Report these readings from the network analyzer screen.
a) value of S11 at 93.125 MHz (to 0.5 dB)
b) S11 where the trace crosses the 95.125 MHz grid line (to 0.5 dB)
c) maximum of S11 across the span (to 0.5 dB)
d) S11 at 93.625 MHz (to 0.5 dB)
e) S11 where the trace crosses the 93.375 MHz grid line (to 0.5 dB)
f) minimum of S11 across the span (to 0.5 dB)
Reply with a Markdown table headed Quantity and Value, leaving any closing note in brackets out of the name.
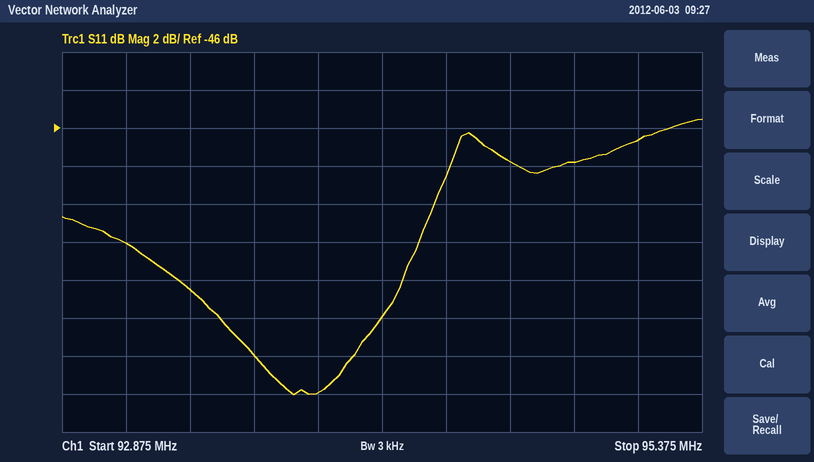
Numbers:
| Quantity | Value |
|---|---|
| value of S11 at 93.125 MHz | -52.0 dB |
| S11 where the trace crosses the 95.125 MHz grid line | -46.5 dB |
| maximum of S11 across the span | -45.5 dB |
| S11 at 93.625 MHz | -58.0 dB |
| S11 where the trace crosses the 93.375 MHz grid line | -54.5 dB |
| minimum of S11 across the span | -60.0 dB |
